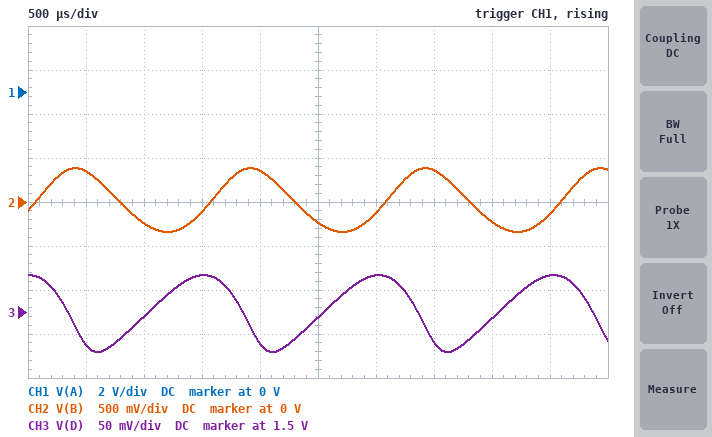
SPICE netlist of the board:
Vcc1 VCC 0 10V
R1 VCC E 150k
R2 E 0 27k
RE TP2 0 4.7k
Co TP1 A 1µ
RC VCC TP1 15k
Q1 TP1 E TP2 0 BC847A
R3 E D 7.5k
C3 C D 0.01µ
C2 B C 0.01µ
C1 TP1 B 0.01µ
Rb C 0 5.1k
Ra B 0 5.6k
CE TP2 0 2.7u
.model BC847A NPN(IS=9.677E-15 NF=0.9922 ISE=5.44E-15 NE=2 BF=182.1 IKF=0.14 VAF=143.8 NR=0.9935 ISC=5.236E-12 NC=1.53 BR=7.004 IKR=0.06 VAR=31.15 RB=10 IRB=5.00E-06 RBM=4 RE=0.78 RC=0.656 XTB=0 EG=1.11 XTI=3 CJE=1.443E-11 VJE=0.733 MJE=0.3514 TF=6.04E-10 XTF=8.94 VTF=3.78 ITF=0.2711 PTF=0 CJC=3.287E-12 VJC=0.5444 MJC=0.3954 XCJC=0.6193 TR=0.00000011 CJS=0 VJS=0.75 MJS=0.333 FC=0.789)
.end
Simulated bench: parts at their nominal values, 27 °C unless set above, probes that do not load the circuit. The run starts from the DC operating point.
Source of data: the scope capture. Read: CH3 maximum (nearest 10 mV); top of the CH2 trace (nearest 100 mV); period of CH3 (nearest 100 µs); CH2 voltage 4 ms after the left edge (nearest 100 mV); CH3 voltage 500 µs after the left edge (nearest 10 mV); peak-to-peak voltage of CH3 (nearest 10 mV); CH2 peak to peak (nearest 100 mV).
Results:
1.54 V
400 mV
1.5 ms
-200 mV
1.46 V
90 mV
700 mV
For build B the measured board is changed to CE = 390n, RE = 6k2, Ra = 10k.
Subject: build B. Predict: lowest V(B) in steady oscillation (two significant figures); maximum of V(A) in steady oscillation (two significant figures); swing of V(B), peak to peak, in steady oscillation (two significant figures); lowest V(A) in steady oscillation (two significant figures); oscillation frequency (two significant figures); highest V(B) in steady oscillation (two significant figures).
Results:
-500 mV
9.2 V
1.0 V
6.3 V
870 Hz
510 mV
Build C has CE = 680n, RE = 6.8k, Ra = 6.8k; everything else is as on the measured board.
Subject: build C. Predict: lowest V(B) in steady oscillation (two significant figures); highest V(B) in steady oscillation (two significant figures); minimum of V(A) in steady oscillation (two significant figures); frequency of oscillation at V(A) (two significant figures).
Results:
-300 mV
320 mV
6.9 V
820 Hz
